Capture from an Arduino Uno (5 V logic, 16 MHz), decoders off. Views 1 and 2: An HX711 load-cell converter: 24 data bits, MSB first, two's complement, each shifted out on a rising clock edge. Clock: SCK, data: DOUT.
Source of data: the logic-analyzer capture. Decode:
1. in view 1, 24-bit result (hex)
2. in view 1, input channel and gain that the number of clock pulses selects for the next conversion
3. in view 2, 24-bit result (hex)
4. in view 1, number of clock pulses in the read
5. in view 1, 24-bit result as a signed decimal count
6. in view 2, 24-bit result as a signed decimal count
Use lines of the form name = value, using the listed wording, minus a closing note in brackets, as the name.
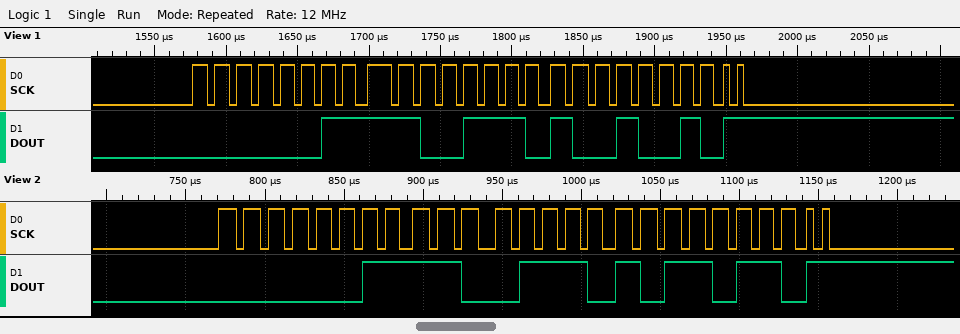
in view 1, 24-bit result = 0x03CE92
in view 1, input channel and gain that the number of clock pulses selects for the next conversion = channel B, gain 32
in view 2, 24-bit result = 0x03CEB6
in view 1, number of clock pulses in the read = 26
in view 1, 24-bit result as a signed decimal count = 249490
in view 2, 24-bit result as a signed decimal count = 249526
